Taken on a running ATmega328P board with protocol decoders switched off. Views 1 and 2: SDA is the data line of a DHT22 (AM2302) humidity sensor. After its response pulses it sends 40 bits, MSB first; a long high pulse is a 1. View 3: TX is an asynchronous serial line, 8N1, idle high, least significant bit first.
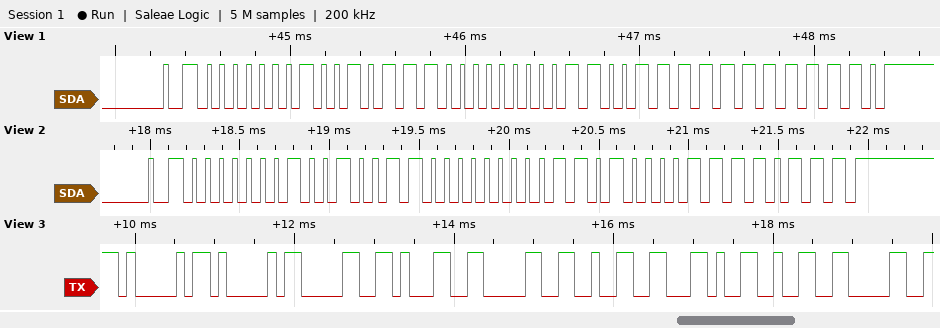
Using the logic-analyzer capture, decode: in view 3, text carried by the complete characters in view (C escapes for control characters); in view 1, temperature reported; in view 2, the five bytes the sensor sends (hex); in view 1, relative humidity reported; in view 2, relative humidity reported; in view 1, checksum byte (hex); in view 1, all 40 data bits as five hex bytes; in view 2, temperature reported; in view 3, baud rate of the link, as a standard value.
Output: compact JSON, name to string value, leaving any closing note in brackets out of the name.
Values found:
{"in view 3, text carried by the complete characters in view": "\"AA0102,20\"", "in view 1, temperature reported": "20.7 °C", "in view 2, the five bytes the sensor sends": "01 26 00 D0 F7", "in view 1, relative humidity reported": "30.2 %", "in view 2, relative humidity reported": "29.4 %", "in view 1, checksum byte": "0xFE", "in view 1, all 40 data bits as five hex bytes": "01 2E 00 CF FE", "in view 2, temperature reported": "20.8 °C", "in view 3, baud rate of the link, as a standard value": "9600 baud"}
